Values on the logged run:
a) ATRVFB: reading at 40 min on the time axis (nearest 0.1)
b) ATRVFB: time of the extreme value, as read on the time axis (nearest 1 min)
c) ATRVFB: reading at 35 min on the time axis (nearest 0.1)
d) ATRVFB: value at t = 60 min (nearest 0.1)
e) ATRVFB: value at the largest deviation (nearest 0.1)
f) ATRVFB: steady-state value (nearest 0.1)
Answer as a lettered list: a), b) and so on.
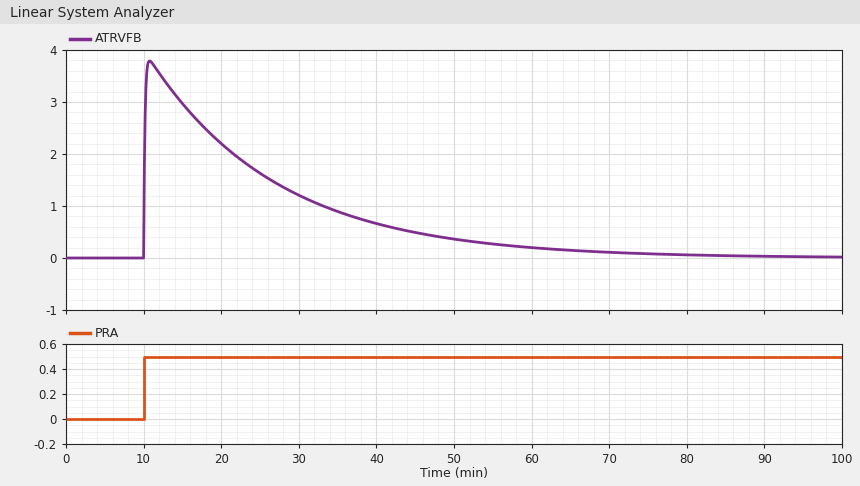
a) 0.7
b) 11 min
c) 0.9
d) 0.2
e) 3.8
f) 0.0
